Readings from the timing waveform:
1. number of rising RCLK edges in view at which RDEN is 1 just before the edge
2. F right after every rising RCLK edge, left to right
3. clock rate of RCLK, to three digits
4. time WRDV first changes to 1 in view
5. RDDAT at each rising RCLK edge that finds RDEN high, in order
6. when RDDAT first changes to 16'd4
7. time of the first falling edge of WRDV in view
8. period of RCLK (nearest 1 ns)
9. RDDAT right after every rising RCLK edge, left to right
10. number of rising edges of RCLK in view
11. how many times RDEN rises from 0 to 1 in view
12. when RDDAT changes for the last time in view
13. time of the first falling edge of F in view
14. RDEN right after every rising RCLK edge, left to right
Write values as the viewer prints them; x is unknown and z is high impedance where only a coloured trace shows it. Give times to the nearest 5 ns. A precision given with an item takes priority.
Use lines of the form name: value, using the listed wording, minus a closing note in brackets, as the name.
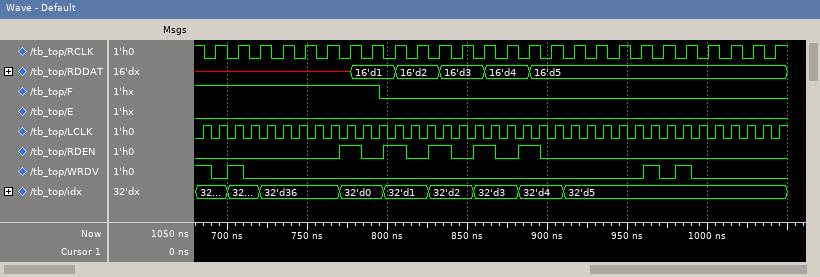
number of rising RCLK edges in view at which RDEN is 1 just before the edge: 5
F right after every rising RCLK edge, left to right: 1 1 1 1 1 1 1 1 0 0 0 0 0 0 0 0 0 0 0 0 0 0 0 0 0 0
clock rate of RCLK, to three digits: 71.4 MHz
time WRDV first changes to 1 in view: 700 ns
RDDAT at each rising RCLK edge that finds RDEN high, in order: x, 16'd1, 16'd2, 16'd3, 16'd4
when RDDAT first changes to 16'd4: 860 ns
time of the first falling edge of WRDV in view: 690 ns
period of RCLK: 14 ns
RDDAT right after every rising RCLK edge, left to right: x, x, x, x, x, x, 16'd1, 16'd1, 16'd2, 16'd2, 16'd3, 16'd3, 16'd4, 16'd4, 16'd5, 16'd5, 16'd5, 16'd5, 16'd5, 16'd5, 16'd5, 16'd5, 16'd5, 16'd5, 16'd5, 16'd5
number of rising edges of RCLK in view: 26
how many times RDEN rises from 0 to 1 in view: 5
when RDDAT changes for the last time in view: 890 ns
time of the first falling edge of F in view: 795 ns
RDEN right after every rising RCLK edge, left to right: 0 0 0 0 0 0 1 0 1 0 1 0 1 0 1 0 0 0 0 0 0 0 0 0 0 0
